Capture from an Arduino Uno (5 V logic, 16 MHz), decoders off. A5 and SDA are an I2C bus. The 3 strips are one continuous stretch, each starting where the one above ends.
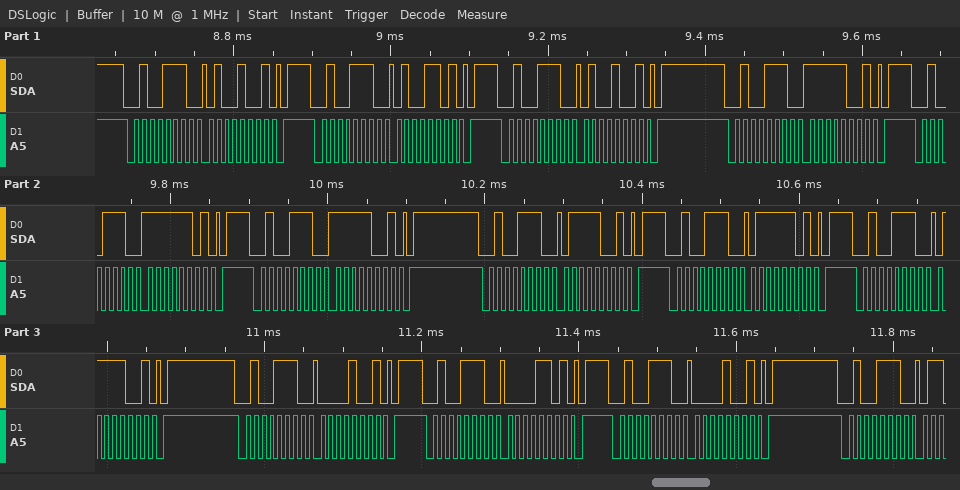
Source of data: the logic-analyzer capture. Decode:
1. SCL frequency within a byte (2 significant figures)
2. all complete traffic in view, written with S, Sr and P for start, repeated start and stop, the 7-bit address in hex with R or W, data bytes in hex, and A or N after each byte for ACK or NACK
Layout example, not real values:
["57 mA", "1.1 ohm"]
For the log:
["100 kHz", "S 27W A 49 A P S 27W A 4D A P S 27W A 49 A P S 27W A F9 A P S 27W A FD A P S 27W A F9 A P S 27W A 79 A P S 27W A 7D A P S 27W A 79 A P S 27W A 09 A P S 27W A 0D A P S 27W A 09 A P S 27W A"]
